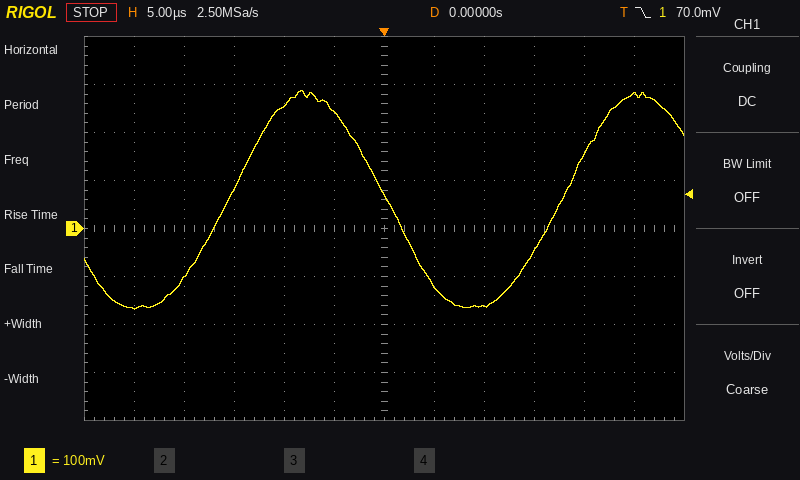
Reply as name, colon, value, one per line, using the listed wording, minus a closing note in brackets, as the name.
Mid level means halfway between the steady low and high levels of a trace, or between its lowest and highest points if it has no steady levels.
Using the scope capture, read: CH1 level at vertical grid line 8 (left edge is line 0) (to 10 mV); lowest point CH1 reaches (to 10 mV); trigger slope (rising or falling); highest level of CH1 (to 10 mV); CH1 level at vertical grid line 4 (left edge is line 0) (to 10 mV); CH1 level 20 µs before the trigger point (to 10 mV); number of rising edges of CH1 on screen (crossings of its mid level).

CH1 level at vertical grid line 8 (left edge is line 0): -160 mV
lowest point CH1 reaches: -170 mV
trigger slope: falling
highest level of CH1: 290 mV
CH1 level at vertical grid line 4 (left edge is line 0): 260 mV
CH1 level 20 µs before the trigger point: -100 mV
number of rising edges of CH1 on screen: 2
